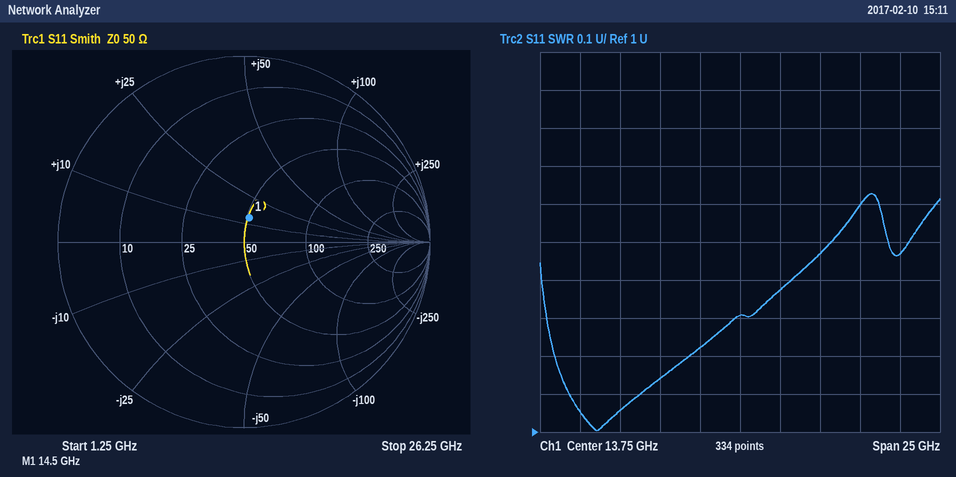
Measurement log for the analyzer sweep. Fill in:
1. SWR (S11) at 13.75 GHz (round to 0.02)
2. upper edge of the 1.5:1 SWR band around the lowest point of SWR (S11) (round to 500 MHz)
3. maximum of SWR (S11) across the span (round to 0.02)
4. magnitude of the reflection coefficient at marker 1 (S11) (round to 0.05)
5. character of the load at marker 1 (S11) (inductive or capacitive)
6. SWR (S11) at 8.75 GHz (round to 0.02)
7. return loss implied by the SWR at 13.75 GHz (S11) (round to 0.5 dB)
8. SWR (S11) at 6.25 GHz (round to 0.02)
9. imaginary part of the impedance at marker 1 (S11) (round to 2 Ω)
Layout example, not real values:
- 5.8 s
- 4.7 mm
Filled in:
- 1.30
- 19.5 GHz
- 1.62
- 0.15
- inductive
- 1.14
- 17.5 dB
- 1.06
- +14 Ω
